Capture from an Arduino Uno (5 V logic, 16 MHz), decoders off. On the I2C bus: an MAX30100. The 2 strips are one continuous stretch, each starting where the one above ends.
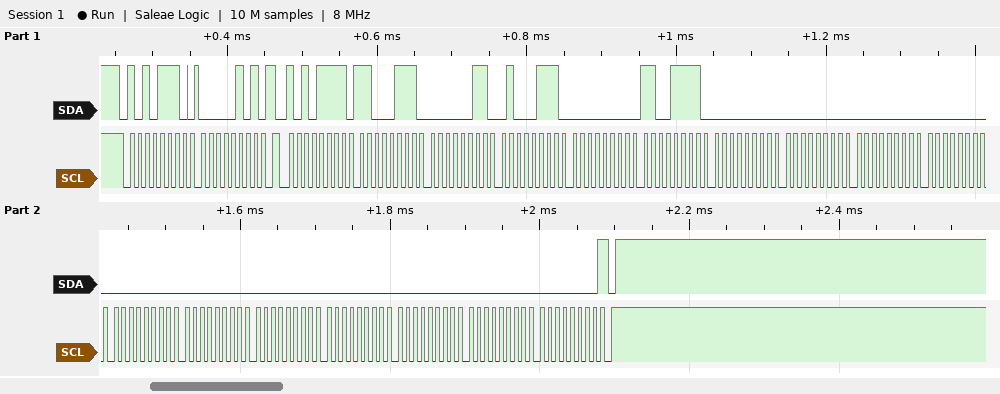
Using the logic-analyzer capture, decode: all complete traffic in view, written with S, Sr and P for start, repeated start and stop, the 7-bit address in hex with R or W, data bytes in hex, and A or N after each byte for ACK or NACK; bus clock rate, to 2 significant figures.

S 57W A 05 A Sr 57R A C7 A 03 A 47 A 00 A CF A 00 A 00 A 00 A 00 A 00 A 00 A 00 A 00 A 00 A 00 A 00 N P
100 kHz
